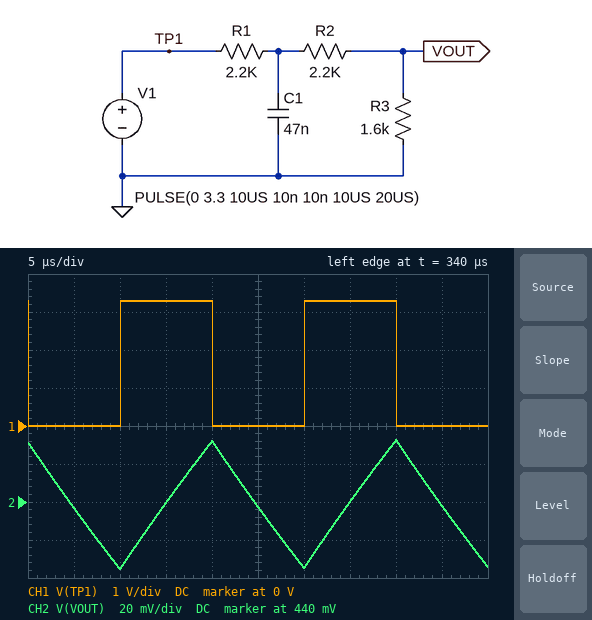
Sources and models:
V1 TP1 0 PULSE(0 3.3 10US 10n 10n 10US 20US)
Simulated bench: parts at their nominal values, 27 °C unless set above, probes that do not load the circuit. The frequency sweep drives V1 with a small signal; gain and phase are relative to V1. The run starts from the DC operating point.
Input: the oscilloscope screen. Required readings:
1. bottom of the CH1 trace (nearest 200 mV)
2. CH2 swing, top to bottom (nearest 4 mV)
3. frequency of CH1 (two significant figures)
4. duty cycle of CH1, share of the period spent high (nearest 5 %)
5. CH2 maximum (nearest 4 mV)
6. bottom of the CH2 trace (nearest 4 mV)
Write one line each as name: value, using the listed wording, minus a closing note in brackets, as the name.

bottom of the CH1 trace: 0 V
CH2 swing, top to bottom: 68 mV
frequency of CH1: 50 kHz
duty cycle of CH1, share of the period spent high: 50 %
CH2 maximum: 472 mV
bottom of the CH2 trace: 404 mV
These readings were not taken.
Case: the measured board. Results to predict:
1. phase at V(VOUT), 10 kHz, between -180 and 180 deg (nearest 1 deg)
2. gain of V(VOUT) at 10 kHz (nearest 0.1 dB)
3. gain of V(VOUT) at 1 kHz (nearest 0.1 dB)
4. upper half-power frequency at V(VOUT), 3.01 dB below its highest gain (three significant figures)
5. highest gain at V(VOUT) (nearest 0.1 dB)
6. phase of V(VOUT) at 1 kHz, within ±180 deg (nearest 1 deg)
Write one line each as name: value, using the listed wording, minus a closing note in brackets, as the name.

phase at V(VOUT), 10 kHz, between -180 and 180 deg: -76 deg
gain of V(VOUT) at 10 kHz: -24.0 dB
gain of V(VOUT) at 1 kHz: -12.2 dB
upper half-power frequency at V(VOUT), 3.01 dB below its highest gain: 2.43 kHz
highest gain at V(VOUT): -11.5 dB
phase of V(VOUT) at 1 kHz, within ±180 deg: -22 deg
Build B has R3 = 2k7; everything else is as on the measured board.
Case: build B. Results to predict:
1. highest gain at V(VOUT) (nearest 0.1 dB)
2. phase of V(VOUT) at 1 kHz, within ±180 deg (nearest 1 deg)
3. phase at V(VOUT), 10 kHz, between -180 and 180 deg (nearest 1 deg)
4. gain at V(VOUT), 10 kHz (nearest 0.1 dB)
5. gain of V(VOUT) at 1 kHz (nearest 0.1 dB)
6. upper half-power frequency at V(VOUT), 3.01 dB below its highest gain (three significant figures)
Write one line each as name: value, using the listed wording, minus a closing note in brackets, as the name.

highest gain at V(VOUT): -8.4 dB
phase of V(VOUT) at 1 kHz, within ±180 deg: -24 deg
phase at V(VOUT), 10 kHz, between -180 and 180 deg: -77 deg
gain at V(VOUT), 10 kHz: -21.6 dB
gain of V(VOUT) at 1 kHz: -9.2 dB
upper half-power frequency at V(VOUT), 3.01 dB below its highest gain: 2.23 kHz
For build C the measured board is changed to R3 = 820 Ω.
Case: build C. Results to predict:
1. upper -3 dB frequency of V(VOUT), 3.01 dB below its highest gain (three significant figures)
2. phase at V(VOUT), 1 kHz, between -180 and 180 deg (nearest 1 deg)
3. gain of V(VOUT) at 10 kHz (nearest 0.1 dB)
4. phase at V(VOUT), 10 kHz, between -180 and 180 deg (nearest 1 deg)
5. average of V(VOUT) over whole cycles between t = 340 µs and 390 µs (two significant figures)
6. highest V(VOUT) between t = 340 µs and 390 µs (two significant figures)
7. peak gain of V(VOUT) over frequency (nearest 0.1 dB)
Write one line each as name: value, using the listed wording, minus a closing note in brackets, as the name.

upper -3 dB frequency of V(VOUT), 3.01 dB below its highest gain: 2.66 kHz
phase at V(VOUT), 1 kHz, between -180 and 180 deg: -21 deg
gain of V(VOUT) at 10 kHz: -27.9 dB
phase at V(VOUT), 10 kHz, between -180 and 180 deg: -75 deg
average of V(VOUT) over whole cycles between t = 340 µs and 390 µs: 260 mV
highest V(VOUT) between t = 340 µs and 390 µs: 280 mV
peak gain of V(VOUT) over frequency: -16.1 dB
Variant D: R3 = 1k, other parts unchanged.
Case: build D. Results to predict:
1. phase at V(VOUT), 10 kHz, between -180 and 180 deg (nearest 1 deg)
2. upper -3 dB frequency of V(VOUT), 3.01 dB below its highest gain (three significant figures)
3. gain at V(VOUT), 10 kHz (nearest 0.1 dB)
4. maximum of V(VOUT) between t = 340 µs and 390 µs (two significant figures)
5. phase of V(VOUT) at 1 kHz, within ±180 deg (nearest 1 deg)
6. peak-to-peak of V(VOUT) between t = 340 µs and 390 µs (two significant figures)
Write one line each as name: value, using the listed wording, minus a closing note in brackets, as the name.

phase at V(VOUT), 10 kHz, between -180 and 180 deg: -75 deg
upper -3 dB frequency of V(VOUT), 3.01 dB below its highest gain: 2.60 kHz
gain at V(VOUT), 10 kHz: -26.6 dB
maximum of V(VOUT) between t = 340 µs and 390 µs: 330 mV
phase of V(VOUT) at 1 kHz, within ±180 deg: -21 deg
peak-to-peak of V(VOUT) between t = 340 µs and 390 µs: 50 mV
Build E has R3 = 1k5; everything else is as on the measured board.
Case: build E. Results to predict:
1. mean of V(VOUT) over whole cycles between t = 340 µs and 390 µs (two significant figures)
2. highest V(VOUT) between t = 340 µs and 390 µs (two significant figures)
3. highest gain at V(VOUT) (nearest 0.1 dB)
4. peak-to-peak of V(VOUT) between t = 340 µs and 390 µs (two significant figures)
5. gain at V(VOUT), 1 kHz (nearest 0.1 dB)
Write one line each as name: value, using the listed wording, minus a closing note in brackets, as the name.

mean of V(VOUT) over whole cycles between t = 340 µs and 390 µs: 420 mV
highest V(VOUT) between t = 340 µs and 390 µs: 450 mV
highest gain at V(VOUT): -11.9 dB
peak-to-peak of V(VOUT) between t = 340 µs and 390 µs: 65 mV
gain at V(VOUT), 1 kHz: -12.6 dB
